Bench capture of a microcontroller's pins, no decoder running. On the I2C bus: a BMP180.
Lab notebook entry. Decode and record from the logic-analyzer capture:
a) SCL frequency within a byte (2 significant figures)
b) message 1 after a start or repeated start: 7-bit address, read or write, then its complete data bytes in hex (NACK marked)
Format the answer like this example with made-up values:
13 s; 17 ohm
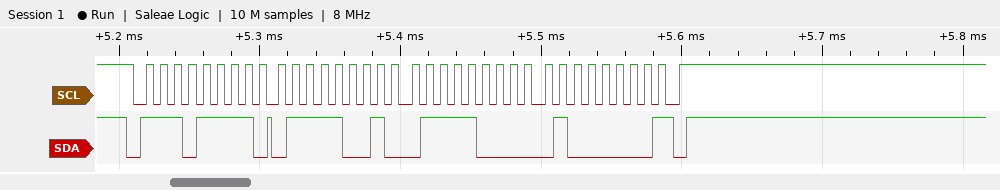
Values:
100 kHz; 0x77 read: 79 78 40 NACK
